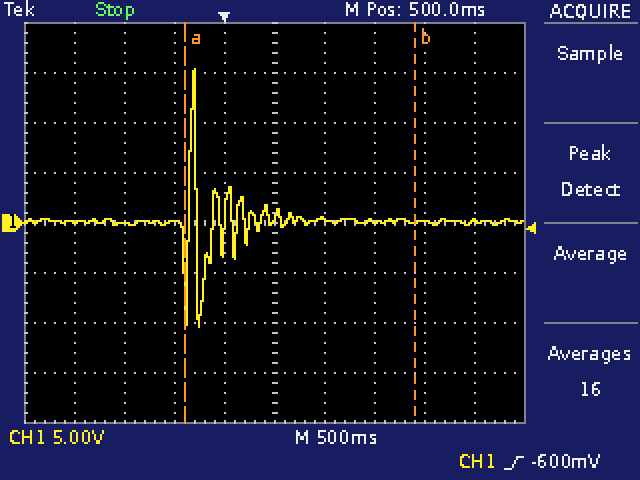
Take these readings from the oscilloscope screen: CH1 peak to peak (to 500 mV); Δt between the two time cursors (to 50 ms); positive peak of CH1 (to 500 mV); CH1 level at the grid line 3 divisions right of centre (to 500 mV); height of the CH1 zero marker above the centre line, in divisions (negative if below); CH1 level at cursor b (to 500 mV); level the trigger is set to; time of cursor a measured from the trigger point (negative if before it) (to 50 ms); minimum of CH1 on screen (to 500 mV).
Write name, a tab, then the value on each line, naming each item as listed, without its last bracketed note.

CH1 peak to peak	26.0 V
Δt between the two time cursors	2.30 s
positive peak of CH1	15.5 V
CH1 level at the grid line 3 divisions right of centre	0.0 V
height of the CH1 zero marker above the centre line, in divisions	0.0 div
CH1 level at cursor b	0.0 V
level the trigger is set to	-600 mV
time of cursor a measured from the trigger point (negative if before it)	-400 ms
minimum of CH1 on screen	-10.5 V
